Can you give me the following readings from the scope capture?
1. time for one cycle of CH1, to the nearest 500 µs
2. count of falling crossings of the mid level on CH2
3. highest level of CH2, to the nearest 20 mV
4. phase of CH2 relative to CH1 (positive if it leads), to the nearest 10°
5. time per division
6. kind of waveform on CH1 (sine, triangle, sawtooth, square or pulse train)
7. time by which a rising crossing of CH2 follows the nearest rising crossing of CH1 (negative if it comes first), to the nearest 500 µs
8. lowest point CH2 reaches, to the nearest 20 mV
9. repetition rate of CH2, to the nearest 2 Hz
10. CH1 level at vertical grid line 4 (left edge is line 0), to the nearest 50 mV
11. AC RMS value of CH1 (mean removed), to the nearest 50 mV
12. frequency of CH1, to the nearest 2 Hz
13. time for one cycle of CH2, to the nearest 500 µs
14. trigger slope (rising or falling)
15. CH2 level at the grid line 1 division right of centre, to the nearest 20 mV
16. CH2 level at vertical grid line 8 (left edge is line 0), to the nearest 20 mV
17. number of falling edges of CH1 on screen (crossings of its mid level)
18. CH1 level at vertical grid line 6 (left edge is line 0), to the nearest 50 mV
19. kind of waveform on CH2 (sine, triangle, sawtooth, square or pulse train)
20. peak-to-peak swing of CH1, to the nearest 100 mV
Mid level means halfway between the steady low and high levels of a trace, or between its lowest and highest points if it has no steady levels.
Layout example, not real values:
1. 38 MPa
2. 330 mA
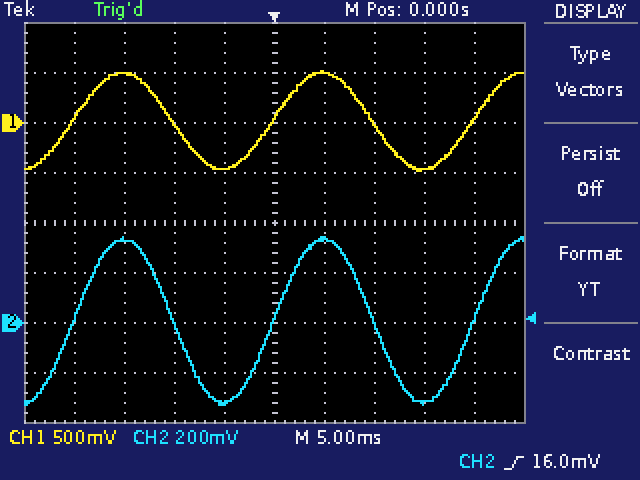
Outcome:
1. 20.0 ms
2. 2
3. 340 mV
4. 0°
5. 5 ms
6. sine
7. 0.0 ms
8. -320 mV
9. 50 Hz
10. -450 mV
11. 350 mV
12. 50 Hz
13. 20.0 ms
14. rising
15. 340 mV
16. -320 mV
17. 2
18. 500 mV
19. sine
20. 1.00 V
